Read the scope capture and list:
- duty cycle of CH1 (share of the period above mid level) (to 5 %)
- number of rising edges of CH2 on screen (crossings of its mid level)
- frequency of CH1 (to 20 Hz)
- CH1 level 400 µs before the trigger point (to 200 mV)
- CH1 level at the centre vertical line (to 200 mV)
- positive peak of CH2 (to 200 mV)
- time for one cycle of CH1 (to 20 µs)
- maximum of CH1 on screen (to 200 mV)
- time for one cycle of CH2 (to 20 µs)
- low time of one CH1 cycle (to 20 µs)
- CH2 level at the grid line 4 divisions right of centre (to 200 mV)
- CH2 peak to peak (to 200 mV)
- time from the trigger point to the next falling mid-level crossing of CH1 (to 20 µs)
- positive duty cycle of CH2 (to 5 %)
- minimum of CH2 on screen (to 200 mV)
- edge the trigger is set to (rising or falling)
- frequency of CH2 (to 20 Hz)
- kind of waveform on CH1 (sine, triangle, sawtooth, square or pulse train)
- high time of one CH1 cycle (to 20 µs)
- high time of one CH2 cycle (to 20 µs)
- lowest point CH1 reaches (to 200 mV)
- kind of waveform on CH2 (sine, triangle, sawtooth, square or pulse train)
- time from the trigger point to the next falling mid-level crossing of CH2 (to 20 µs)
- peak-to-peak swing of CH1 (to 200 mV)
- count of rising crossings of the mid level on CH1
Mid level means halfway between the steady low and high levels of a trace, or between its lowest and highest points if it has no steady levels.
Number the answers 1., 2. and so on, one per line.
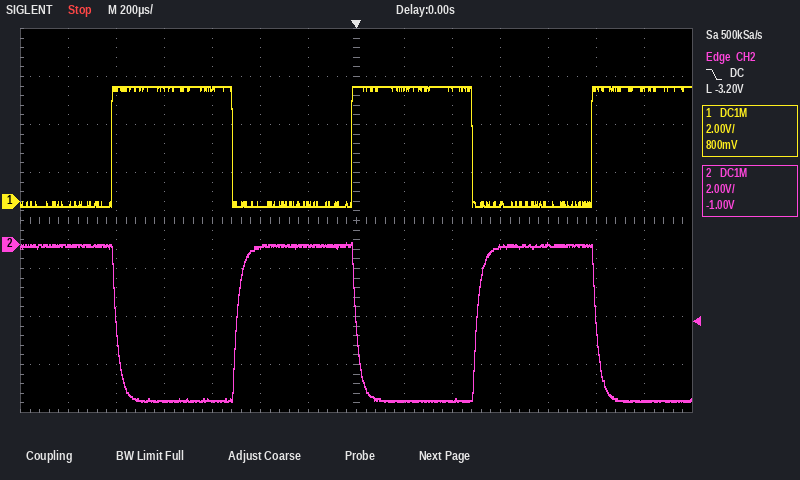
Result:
1. 50 %
2. 2
3. 1.00 kHz
4. -200 mV
5. 4.8 V
6. 0.0 V
7. 1.00 ms
8. 4.8 V
9. 1.00 ms
10. 500 µs
11. 0.0 V
12. 6.6 V
13. 480 µs
14. 50 %
15. -6.6 V
16. falling
17. 1.00 kHz
18. square
19. 500 µs
20. 500 µs
21. -200 mV
22. square
23. 1.00 ms
24. 5.0 V
25. 3
